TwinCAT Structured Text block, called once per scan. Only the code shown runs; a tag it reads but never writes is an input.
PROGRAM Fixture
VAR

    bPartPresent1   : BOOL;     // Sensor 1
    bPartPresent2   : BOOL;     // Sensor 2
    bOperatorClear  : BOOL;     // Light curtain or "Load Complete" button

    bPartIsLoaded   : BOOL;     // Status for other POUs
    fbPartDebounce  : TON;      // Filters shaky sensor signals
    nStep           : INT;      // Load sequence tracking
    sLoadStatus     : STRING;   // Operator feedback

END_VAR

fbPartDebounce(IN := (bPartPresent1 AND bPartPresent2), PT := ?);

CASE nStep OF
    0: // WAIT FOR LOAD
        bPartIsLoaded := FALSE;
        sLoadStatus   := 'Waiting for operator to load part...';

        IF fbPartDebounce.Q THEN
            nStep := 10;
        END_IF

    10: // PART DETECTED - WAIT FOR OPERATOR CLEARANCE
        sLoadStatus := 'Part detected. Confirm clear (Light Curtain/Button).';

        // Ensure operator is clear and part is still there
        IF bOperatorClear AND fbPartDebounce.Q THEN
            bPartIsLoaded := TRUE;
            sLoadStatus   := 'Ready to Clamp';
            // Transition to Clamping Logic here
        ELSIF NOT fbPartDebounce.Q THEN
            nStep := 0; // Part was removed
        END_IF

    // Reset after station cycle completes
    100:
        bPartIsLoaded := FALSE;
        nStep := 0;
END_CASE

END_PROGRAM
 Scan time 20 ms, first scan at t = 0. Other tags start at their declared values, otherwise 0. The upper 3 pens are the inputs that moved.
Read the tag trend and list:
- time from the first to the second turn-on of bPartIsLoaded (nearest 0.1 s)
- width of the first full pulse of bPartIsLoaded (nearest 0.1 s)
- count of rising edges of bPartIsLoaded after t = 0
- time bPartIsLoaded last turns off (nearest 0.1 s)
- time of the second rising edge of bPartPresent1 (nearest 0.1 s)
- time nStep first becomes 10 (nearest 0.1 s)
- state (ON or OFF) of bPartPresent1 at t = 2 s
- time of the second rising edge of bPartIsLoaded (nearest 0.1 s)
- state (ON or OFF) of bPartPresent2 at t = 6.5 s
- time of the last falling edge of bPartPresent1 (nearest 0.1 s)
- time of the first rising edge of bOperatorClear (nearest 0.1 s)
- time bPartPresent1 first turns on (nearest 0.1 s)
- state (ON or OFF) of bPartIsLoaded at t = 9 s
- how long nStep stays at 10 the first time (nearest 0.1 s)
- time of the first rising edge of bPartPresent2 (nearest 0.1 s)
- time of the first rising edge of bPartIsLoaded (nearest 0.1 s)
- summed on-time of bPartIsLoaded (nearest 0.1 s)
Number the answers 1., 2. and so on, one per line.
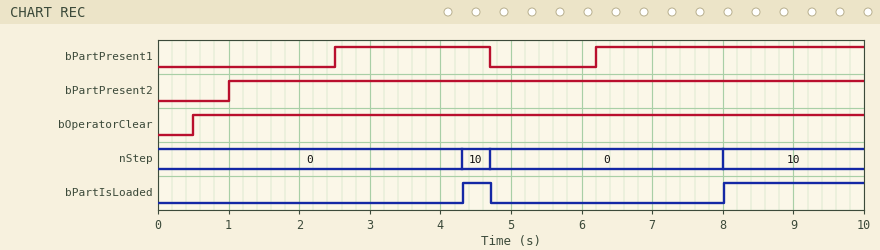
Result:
1. 3.7 s
2. 0.4 s
3. 2
4. 4.7 s
5. 6.2 s
6. 4.3 s
7. OFF
8. 8.0 s
9. ON
10. 4.7 s
11. 0.5 s
12. 2.5 s
13. ON
14. 0.4 s
15. 1.0 s
16. 4.3 s
17. 2.4 s
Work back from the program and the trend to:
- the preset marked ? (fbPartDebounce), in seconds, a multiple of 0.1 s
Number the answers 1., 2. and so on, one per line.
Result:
1. 1.8 s
